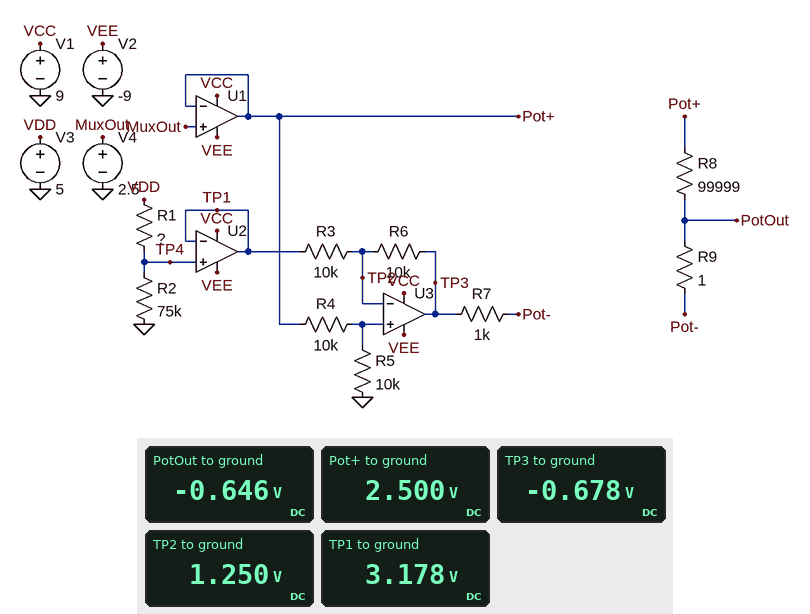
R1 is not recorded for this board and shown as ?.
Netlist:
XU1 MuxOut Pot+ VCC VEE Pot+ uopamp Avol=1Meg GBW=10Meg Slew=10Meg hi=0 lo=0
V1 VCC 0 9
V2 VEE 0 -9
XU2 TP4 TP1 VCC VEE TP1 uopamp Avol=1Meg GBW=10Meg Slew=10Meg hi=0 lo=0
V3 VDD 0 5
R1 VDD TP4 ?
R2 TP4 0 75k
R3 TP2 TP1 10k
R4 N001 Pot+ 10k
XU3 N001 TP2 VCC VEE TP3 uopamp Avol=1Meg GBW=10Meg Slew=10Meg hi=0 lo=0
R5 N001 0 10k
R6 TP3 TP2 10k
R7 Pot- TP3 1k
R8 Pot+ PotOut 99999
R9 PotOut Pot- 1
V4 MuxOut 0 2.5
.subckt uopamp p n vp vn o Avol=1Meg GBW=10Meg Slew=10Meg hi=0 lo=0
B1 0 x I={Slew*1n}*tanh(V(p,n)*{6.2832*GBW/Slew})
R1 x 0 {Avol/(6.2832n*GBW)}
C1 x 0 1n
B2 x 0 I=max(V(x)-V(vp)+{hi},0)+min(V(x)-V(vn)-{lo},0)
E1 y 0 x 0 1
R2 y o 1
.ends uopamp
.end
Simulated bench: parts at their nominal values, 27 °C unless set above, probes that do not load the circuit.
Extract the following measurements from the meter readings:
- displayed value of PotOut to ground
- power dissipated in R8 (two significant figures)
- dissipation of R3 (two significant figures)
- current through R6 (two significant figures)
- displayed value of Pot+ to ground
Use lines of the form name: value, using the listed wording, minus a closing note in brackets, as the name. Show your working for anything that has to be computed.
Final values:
displayed value of PotOut to ground: -0.646 V
power dissipated in R8: (2.5 V - (-646 mV))^2 / 100 kΩ = 99 µW
dissipation of R3: (3.178 V - 1.25 V)^2 / 10 kΩ = 370 µW
current through R6: (1.25 V - (-678 mV)) / 10 kΩ = 190 µA
displayed value of Pot+ to ground: 2.500 V
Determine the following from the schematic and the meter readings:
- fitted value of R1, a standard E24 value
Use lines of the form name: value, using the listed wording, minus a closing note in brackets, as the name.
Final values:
fitted value of R1, a standard E24 value: 43 kΩ
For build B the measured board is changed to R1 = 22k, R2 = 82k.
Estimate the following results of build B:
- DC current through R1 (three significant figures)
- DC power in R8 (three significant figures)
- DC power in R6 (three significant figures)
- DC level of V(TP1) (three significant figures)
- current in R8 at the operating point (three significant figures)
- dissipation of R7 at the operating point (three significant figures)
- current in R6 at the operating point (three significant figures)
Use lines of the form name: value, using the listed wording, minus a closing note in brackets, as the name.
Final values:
DC current through R1: 48.1 µA
DC power in R8: 152 µW
DC power in R6: 725 µW
DC level of V(TP1): 3.94 V
current in R8 at the operating point: 39.0 µA
dissipation of R7 at the operating point: 1.52 µW
current in R6 at the operating point: 269 µA
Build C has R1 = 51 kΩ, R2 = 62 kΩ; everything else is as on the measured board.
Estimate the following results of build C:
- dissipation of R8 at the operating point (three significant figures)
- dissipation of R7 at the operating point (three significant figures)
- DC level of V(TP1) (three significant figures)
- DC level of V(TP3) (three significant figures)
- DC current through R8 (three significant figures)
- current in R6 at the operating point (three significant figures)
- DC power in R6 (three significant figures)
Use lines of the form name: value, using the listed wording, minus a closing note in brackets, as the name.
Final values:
dissipation of R8 at the operating point: 73.8 µW
dissipation of R7 at the operating point: 738 nW
DC level of V(TP1): 2.74 V
DC level of V(TP3): -243 mV
DC current through R8: 27.2 µA
current in R6 at the operating point: 149 µA
DC power in R6: 223 µW
